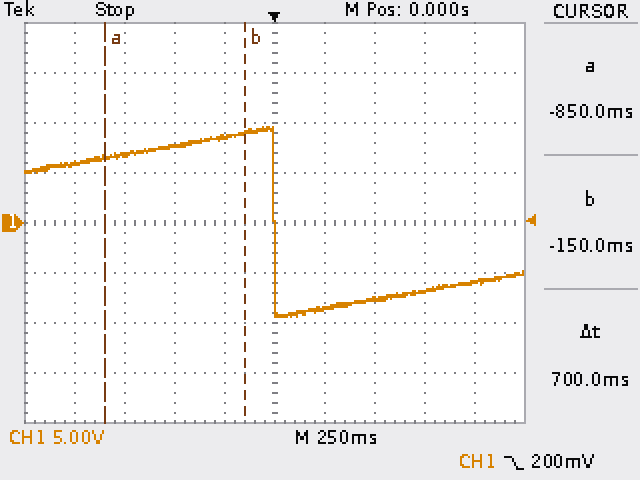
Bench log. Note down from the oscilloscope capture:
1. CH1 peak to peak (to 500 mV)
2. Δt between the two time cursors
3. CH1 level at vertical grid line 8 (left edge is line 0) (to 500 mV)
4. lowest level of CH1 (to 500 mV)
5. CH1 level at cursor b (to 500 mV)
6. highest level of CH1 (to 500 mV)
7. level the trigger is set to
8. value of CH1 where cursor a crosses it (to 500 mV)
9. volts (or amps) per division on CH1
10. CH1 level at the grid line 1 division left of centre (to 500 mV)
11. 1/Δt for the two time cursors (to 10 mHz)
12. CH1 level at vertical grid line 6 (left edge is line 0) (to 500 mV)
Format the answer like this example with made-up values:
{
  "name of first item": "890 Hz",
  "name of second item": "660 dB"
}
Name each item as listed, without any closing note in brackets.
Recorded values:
{
  "CH1 peak to peak": "19.0 V",
  "Δt between the two time cursors": "700 ms",
  "CH1 level at vertical grid line 8 (left edge is line 0)": "-7.0 V",
  "lowest level of CH1": "-9.5 V",
  "CH1 level at cursor b": "9.0 V",
  "highest level of CH1": "9.5 V",
  "level the trigger is set to": "200 mV",
  "value of CH1 where cursor a crosses it": "6.5 V",
  "volts (or amps) per division on CH1": "5 V",
  "CH1 level at the grid line 1 division left of centre": "8.5 V",
  "1/Δt for the two time cursors": "1.43 Hz",
  "CH1 level at vertical grid line 6 (left edge is line 0)": "-8.5 V"
}
